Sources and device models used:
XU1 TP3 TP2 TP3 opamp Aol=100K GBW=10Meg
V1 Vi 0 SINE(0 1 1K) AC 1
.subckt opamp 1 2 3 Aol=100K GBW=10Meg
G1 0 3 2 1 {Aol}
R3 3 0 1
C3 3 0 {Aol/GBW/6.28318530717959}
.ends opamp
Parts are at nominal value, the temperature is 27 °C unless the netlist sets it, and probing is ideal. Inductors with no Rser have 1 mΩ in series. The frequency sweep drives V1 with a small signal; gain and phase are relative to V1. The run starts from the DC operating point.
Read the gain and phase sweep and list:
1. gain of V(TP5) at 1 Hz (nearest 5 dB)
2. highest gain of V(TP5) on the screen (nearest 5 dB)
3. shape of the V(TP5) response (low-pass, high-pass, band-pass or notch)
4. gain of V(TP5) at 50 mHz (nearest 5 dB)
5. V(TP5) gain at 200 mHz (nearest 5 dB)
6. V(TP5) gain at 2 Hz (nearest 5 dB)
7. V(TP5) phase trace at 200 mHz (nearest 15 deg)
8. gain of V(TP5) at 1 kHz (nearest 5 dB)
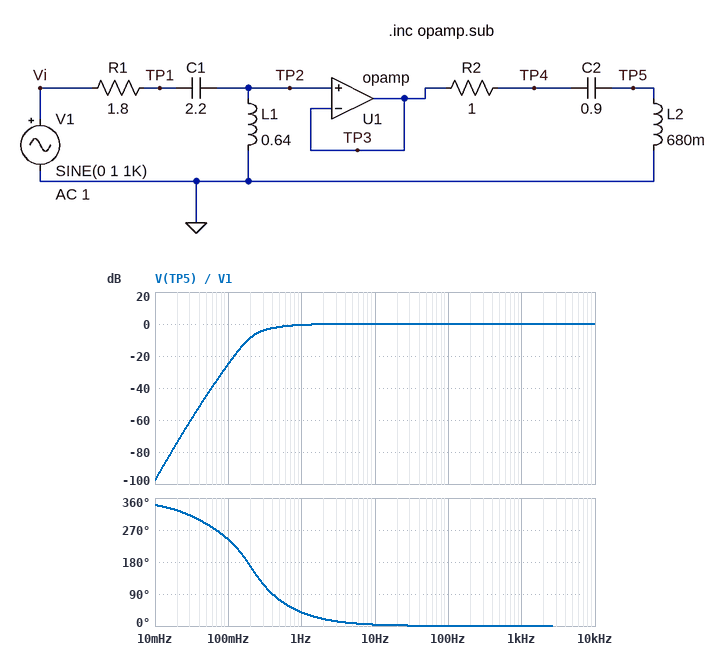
0 dB
0 dB
high-pass
-45 dB
-10 dB
0 dB
165 deg
0 dB
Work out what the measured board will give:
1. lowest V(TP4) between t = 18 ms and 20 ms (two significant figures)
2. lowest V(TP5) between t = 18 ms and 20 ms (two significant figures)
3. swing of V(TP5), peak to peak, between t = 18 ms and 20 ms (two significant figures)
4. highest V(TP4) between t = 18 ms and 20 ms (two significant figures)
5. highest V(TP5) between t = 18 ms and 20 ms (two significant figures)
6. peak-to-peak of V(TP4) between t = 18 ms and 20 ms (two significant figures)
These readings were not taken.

-1.0 V
-1.0 V
2.0 V
1.0 V
1.0 V
2.0 V
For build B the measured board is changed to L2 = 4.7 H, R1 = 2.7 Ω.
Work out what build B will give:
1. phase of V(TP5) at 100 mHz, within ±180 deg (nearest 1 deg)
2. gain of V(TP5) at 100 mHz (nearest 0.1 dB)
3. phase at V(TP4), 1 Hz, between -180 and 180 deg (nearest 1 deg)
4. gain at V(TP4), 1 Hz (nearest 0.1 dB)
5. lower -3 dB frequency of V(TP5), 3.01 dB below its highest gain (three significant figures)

137 deg
-11.0 dB
36 deg
-1.5 dB
628 mHz
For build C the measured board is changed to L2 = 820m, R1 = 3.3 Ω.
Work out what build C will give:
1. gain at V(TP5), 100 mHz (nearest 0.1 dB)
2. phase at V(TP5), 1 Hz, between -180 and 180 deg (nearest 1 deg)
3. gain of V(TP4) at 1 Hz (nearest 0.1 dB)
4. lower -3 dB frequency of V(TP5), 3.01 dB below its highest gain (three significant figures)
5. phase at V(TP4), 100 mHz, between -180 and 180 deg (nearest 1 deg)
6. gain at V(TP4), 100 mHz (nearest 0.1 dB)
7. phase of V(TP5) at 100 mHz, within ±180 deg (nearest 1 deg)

-28.2 dB
51 deg
-2.3 dB
760 mHz
57 deg
-20.5 dB
-123 deg
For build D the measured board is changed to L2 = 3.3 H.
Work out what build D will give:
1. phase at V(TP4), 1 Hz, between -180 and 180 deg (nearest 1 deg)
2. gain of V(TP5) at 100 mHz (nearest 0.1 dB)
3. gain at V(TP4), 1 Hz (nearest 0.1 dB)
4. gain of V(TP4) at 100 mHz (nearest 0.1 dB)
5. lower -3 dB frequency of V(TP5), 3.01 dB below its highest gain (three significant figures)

27 deg
-7.2 dB
-0.7 dB
-23.9 dB
368 mHz
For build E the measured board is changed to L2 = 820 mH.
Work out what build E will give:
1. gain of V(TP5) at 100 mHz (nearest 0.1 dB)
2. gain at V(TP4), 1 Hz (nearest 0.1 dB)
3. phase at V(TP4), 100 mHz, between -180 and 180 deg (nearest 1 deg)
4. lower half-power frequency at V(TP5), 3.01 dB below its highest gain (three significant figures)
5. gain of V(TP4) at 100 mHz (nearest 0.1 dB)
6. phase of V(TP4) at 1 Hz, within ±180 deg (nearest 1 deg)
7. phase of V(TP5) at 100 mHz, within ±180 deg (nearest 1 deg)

-23.0 dB
-0.8 dB
61 deg
342 mHz
-15.3 dB
36 deg
-119 deg
